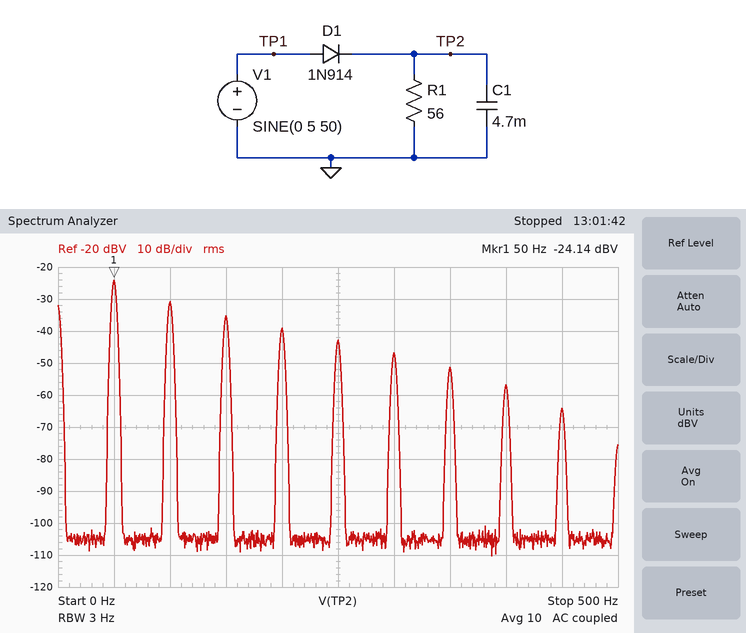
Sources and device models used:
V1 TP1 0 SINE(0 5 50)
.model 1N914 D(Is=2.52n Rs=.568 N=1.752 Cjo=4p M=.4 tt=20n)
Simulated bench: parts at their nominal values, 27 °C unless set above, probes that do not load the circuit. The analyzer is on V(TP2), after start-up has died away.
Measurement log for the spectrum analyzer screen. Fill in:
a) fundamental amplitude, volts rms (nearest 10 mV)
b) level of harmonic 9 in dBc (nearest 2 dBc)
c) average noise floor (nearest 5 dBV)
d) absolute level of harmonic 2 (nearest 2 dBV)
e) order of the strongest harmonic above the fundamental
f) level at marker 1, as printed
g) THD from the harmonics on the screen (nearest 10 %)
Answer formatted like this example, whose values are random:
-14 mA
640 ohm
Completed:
60 mV
-40 dBc
-105 dBV
-30 dBV
2
-24.14 dBV
60 %
